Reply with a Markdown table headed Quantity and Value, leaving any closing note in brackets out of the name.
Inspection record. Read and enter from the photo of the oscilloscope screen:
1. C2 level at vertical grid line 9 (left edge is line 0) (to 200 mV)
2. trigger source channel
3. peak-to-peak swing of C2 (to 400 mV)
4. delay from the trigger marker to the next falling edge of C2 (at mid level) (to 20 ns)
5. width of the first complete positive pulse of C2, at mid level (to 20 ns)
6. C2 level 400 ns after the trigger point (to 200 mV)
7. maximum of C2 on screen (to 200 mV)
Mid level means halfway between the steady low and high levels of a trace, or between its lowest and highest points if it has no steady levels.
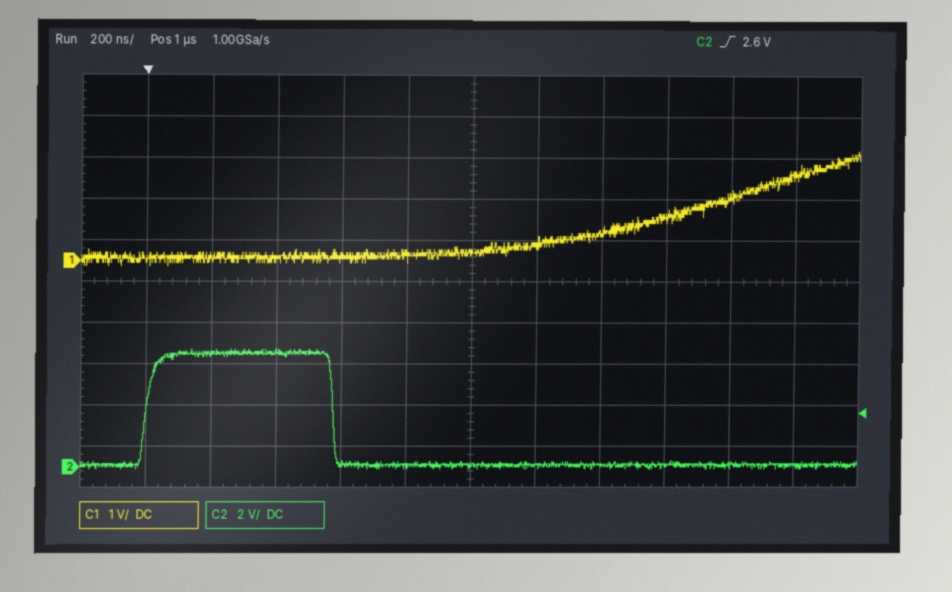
| Quantity | Value |
|---|---|
| C2 level at vertical grid line 9 (left edge is line 0) | 0.0 V |
| trigger source channel | C2 |
| peak-to-peak swing of C2 | 5.6 V |
| delay from the trigger marker to the next falling edge of C2 (at mid level) | 580 ns |
| width of the first complete positive pulse of C2, at mid level | 580 ns |
| C2 level 400 ns after the trigger point | 5.6 V |
| maximum of C2 on screen | 5.6 V |
